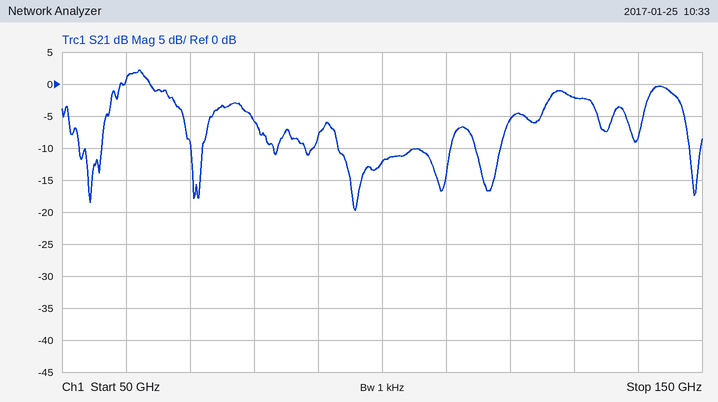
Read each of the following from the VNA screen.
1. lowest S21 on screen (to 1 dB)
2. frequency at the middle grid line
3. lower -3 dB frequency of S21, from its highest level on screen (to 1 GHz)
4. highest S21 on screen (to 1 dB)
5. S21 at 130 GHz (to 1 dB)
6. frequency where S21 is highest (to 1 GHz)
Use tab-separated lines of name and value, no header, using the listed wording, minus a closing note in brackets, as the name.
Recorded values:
lowest S21 on screen	-20 dB
frequency at the middle grid line	100 GHz
lower -3 dB frequency of S21, from its highest level on screen	59 GHz
highest S21 on screen	2 dB
S21 at 130 GHz	-2 dB
frequency where S21 is highest	62 GHz
